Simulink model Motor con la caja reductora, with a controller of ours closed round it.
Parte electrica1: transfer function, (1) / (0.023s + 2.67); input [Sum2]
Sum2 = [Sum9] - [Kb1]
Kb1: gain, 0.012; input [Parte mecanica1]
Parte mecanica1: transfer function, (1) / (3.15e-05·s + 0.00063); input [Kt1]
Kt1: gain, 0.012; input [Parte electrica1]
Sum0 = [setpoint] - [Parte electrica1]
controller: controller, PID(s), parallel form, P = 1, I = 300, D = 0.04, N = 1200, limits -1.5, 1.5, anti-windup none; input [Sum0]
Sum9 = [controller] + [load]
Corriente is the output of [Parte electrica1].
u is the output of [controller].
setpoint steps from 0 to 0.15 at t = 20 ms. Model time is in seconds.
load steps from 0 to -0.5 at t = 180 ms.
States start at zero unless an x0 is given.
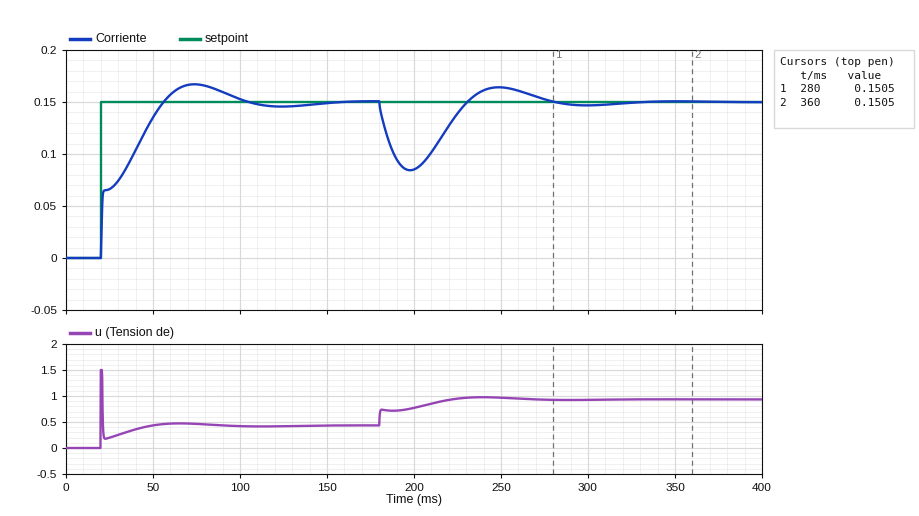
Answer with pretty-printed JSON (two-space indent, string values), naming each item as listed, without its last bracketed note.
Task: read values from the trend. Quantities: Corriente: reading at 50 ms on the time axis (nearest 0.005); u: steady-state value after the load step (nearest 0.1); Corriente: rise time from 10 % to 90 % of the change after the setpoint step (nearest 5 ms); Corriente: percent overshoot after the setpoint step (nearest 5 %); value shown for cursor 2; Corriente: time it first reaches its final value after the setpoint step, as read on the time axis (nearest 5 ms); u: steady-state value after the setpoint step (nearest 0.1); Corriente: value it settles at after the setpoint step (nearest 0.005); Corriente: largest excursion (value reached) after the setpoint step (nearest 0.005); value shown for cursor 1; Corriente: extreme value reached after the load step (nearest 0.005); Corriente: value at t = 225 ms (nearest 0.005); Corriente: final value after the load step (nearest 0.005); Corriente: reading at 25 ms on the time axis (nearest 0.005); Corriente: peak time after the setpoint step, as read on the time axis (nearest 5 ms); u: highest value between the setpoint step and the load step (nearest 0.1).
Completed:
{
  "Corriente: reading at 50 ms on the time axis": "0.135",
  "u: steady-state value after the load step": "0.9",
  "Corriente: rise time from 10 % to 90 % of the change after the setpoint step": "30 ms",
  "Corriente: percent overshoot after the setpoint step": "10 %",
  "value shown for cursor 2": "0.1505",
  "Corriente: time it first reaches its final value after the setpoint step, as read on the time axis": "55 ms",
  "u: steady-state value after the setpoint step": "0.4",
  "Corriente: value it settles at after the setpoint step": "0.150",
  "Corriente: largest excursion (value reached) after the setpoint step": "0.165",
  "value shown for cursor 1": "0.1505",
  "Corriente: extreme value reached after the load step": "0.085",
  "Corriente: value at t = 225 ms": "0.140",
  "Corriente: final value after the load step": "0.150",
  "Corriente: reading at 25 ms on the time axis": "0.065",
  "Corriente: peak time after the setpoint step, as read on the time axis": "75 ms",
  "u: highest value between the setpoint step and the load step": "1.5"
}
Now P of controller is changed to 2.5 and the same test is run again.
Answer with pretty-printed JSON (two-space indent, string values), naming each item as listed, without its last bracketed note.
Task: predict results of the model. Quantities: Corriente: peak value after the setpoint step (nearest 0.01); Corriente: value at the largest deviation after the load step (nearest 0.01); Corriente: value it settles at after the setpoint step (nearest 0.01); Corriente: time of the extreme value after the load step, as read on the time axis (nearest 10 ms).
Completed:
{
  "Corriente: peak value after the setpoint step": "0.16",
  "Corriente: value at the largest deviation after the load step": "0.09",
  "Corriente: value it settles at after the setpoint step": "0.15",
  "Corriente: time of the extreme value after the load step, as read on the time axis": "200 ms"
}
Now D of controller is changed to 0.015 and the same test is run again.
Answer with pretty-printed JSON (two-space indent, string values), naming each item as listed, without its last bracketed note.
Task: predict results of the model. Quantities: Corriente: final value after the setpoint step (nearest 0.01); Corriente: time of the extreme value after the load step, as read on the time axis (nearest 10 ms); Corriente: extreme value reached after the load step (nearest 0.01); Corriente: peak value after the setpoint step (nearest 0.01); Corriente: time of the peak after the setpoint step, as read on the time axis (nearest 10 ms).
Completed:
{
  "Corriente: final value after the setpoint step": "0.15",
  "Corriente: time of the extreme value after the load step, as read on the time axis": "190 ms",
  "Corriente: extreme value reached after the load step": "0.07",
  "Corriente: peak value after the setpoint step": "0.16",
  "Corriente: time of the peak after the setpoint step, as read on the time axis": "60 ms"
}
